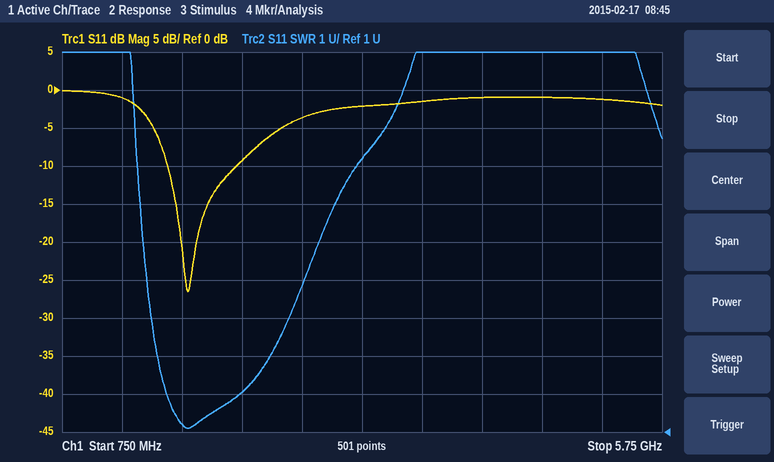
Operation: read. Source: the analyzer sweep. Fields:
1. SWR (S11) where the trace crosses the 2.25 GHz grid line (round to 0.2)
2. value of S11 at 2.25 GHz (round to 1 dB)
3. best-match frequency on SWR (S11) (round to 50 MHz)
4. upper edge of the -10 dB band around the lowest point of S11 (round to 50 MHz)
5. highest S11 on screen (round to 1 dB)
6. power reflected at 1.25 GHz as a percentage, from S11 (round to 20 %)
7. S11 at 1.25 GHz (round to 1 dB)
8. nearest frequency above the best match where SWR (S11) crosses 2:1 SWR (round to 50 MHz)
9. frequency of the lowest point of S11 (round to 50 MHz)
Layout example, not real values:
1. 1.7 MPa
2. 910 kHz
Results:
1. 2.0
2. -9 dB
3. 1.80 GHz
4. 2.20 GHz
5. 0 dB
6. 80 %
7. -1 dB
8. 2.25 GHz
9. 1.80 GHz
